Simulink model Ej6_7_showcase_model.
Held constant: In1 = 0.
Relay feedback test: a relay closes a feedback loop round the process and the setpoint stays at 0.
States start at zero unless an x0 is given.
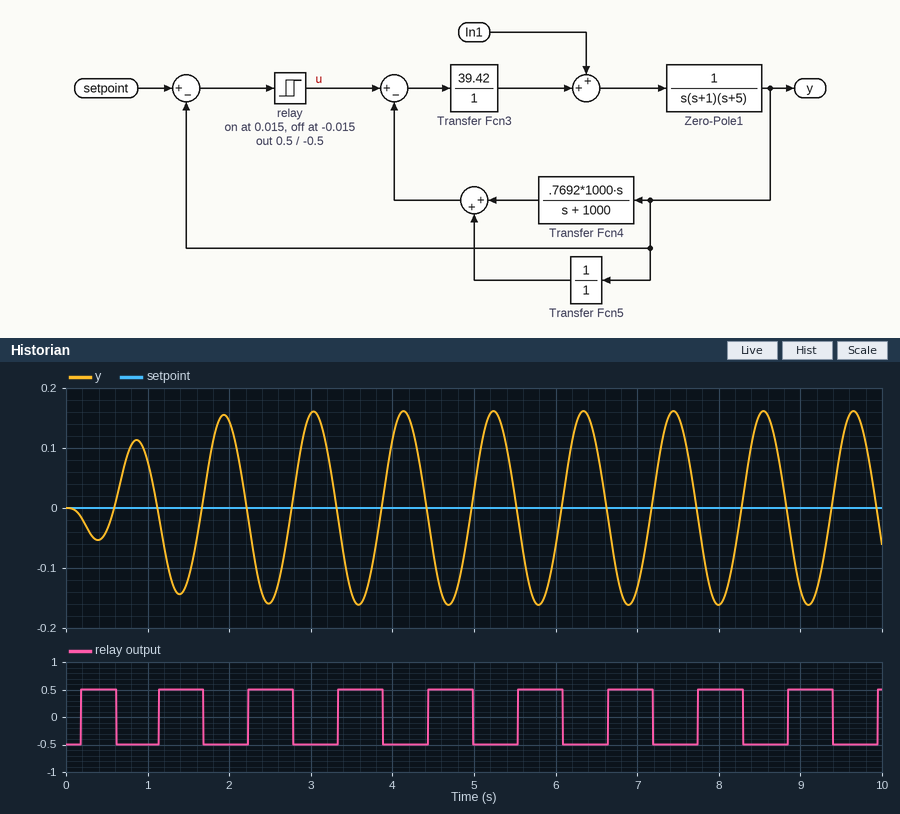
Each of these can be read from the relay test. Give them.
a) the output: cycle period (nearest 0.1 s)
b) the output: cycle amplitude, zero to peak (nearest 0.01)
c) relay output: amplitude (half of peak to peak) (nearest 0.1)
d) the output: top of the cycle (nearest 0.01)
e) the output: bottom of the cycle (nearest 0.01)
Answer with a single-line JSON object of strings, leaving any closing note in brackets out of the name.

{"the output: cycle period": "1.1 s", "the output: cycle amplitude, zero to peak": "0.16", "relay output: amplitude (half of peak to peak)": "0.5", "the output: top of the cycle": "0.16", "the output: bottom of the cycle": "-0.16"}
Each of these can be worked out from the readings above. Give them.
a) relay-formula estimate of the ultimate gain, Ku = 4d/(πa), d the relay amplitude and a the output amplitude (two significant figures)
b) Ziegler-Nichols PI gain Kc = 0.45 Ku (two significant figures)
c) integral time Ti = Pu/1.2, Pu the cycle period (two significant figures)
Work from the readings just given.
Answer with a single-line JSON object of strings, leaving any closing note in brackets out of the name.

{"relay-formula estimate of the ultimate gain, Ku = 4d/(πa), d the relay amplitude and a the output amplitude": "4.0", "Ziegler-Nichols PI gain Kc = 0.45 Ku": "1.8", "integral time Ti = Pu/1.2, Pu the cycle period": "0.92 s"}
